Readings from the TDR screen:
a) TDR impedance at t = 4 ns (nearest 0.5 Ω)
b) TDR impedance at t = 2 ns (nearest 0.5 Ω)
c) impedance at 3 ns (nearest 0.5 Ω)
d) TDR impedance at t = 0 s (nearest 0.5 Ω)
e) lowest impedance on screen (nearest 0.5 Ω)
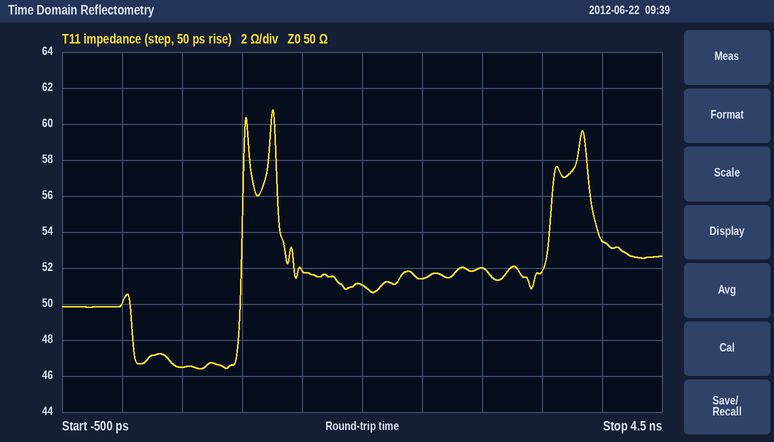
53.5 Ω
51.0 Ω
52.0 Ω
50.0 Ω
46.5 Ω
